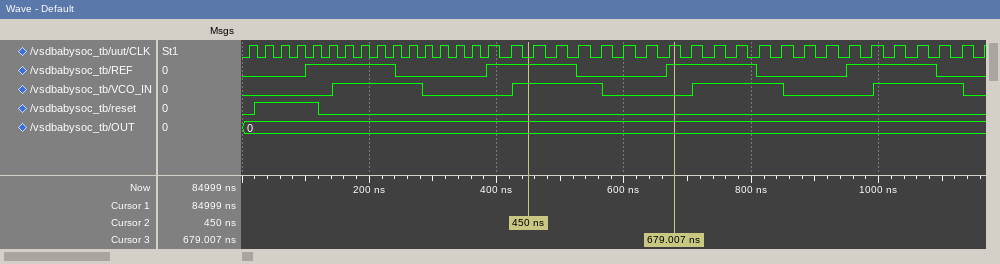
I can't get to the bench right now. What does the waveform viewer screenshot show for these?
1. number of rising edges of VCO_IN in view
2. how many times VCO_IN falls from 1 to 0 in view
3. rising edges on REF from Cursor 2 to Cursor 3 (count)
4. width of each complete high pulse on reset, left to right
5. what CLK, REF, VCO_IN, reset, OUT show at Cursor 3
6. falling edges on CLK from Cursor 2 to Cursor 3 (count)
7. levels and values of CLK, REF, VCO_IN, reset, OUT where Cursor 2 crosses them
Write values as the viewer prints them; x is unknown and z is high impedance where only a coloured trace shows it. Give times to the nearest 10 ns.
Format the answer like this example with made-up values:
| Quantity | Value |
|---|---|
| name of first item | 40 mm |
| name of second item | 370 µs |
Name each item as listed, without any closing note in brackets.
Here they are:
| Quantity | Value |
|---|---|
| number of rising edges of VCO_IN in view | 4 |
| how many times VCO_IN falls from 1 to 0 in view | 4 |
| rising edges on REF from Cursor 2 to Cursor 3 | 1 |
| width of each complete high pulse on reset, left to right | 100 ns |
| what CLK, REF, VCO_IN, reset, OUT show at Cursor 3 | CLK=1, REF=1, VCO_IN=0, reset=0, OUT=0 |
| falling edges on CLK from Cursor 2 to Cursor 3 | 6 |
| levels and values of CLK, REF, VCO_IN, reset, OUT where Cursor 2 crosses them | CLK=0, REF=1, VCO_IN=1, reset=0, OUT=0 |
